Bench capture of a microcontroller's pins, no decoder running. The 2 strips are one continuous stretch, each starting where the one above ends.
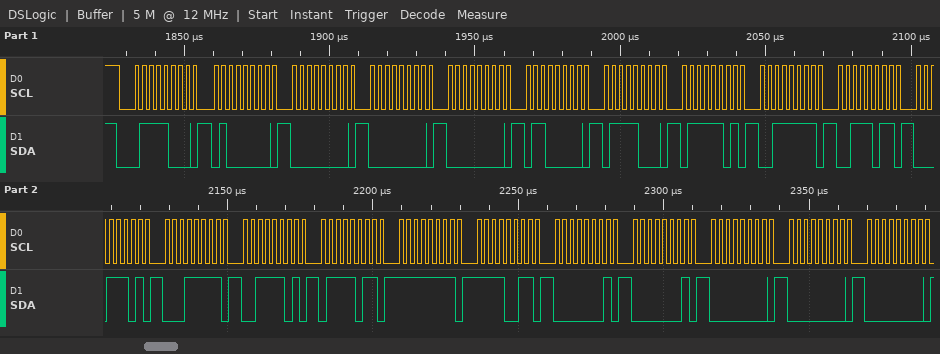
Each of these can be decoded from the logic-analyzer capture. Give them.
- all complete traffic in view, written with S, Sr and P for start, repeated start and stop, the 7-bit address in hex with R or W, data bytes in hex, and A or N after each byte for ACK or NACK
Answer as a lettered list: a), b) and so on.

a) S 3CW A 40 A 00 A 00 A 00 A 60 A 78 A 7D A 3F A 3B A 1D A 1F A 3D A 7B A FF A F3 A 01 A 01 A 00 A 00 A 00 A
